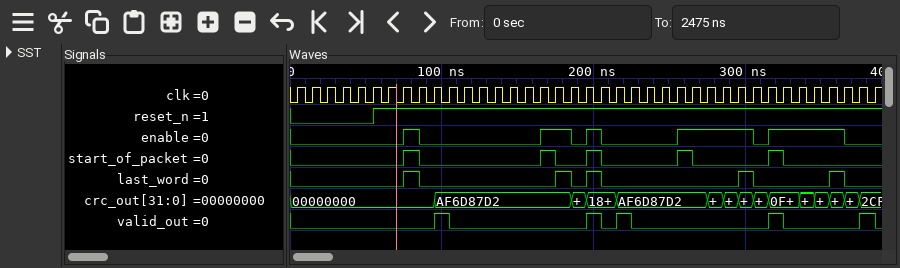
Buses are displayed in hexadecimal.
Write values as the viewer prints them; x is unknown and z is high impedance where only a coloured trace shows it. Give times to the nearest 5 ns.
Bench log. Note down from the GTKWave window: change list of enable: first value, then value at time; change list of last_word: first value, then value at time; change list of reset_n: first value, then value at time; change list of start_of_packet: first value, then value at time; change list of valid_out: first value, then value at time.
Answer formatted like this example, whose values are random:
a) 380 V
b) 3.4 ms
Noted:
a) 0, 1 at 75 ns, 0 at 85 ns, 1 at 165 ns, 0 at 185 ns, 1 at 195 ns, 0 at 205 ns, 1 at 255 ns, 0 at 305 ns, 1 at 315 ns, 0 at 365 ns
b) 0, 1 at 75 ns, 0 at 85 ns, 1 at 175 ns, 0 at 185 ns, 1 at 195 ns, 0 at 205 ns, 1 at 295 ns, 0 at 305 ns, 1 at 355 ns, 0 at 365 ns
c) 0, 1 at 55 ns
d) 0, 1 at 75 ns, 0 at 85 ns, 1 at 165 ns, 0 at 175 ns, 1 at 195 ns, 0 at 205 ns, 1 at 255 ns, 0 at 265 ns, 1 at 315 ns, 0 at 325 ns
e) 0, 1 at 95 ns, 0 at 105 ns, 1 at 195 ns, 0 at 205 ns, 1 at 215 ns, 0 at 225 ns, 1 at 315 ns, 0 at 325 ns, 1 at 375 ns, 0 at 385 ns
